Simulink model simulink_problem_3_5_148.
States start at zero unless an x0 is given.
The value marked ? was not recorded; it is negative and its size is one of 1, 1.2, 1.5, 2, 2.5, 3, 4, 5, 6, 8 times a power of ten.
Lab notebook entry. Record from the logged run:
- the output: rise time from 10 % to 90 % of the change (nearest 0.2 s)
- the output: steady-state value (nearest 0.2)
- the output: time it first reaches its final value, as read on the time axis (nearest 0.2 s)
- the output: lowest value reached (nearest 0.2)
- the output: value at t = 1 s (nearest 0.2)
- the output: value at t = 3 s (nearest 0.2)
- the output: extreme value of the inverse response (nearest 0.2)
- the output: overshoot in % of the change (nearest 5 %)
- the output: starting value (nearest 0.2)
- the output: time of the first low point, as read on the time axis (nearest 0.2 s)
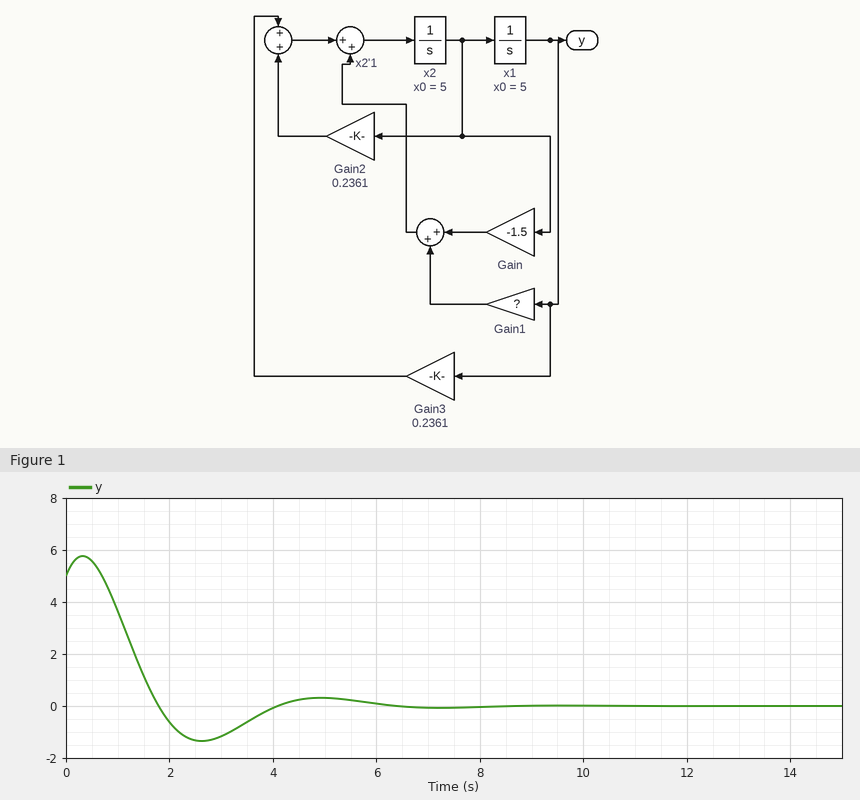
0.8 s
0.0
1.8 s
-1.4
3.6
-1.2
5.8
25 %
5.0
2.6 s
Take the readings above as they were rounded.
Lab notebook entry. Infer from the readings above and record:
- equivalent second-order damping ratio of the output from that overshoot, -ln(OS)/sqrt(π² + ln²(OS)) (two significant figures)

0.40
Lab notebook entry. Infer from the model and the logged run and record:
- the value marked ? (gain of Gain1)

-2.5
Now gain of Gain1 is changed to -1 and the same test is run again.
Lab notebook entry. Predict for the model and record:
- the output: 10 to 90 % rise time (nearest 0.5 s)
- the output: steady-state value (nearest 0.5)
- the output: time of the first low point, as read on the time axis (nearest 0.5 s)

2.0 s
0.0
6.0 s
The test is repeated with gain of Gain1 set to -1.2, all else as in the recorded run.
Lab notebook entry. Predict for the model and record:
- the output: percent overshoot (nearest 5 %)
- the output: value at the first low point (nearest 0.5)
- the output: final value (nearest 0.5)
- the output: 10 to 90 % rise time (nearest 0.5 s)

10 %
-0.5
0.0
1.5 s
